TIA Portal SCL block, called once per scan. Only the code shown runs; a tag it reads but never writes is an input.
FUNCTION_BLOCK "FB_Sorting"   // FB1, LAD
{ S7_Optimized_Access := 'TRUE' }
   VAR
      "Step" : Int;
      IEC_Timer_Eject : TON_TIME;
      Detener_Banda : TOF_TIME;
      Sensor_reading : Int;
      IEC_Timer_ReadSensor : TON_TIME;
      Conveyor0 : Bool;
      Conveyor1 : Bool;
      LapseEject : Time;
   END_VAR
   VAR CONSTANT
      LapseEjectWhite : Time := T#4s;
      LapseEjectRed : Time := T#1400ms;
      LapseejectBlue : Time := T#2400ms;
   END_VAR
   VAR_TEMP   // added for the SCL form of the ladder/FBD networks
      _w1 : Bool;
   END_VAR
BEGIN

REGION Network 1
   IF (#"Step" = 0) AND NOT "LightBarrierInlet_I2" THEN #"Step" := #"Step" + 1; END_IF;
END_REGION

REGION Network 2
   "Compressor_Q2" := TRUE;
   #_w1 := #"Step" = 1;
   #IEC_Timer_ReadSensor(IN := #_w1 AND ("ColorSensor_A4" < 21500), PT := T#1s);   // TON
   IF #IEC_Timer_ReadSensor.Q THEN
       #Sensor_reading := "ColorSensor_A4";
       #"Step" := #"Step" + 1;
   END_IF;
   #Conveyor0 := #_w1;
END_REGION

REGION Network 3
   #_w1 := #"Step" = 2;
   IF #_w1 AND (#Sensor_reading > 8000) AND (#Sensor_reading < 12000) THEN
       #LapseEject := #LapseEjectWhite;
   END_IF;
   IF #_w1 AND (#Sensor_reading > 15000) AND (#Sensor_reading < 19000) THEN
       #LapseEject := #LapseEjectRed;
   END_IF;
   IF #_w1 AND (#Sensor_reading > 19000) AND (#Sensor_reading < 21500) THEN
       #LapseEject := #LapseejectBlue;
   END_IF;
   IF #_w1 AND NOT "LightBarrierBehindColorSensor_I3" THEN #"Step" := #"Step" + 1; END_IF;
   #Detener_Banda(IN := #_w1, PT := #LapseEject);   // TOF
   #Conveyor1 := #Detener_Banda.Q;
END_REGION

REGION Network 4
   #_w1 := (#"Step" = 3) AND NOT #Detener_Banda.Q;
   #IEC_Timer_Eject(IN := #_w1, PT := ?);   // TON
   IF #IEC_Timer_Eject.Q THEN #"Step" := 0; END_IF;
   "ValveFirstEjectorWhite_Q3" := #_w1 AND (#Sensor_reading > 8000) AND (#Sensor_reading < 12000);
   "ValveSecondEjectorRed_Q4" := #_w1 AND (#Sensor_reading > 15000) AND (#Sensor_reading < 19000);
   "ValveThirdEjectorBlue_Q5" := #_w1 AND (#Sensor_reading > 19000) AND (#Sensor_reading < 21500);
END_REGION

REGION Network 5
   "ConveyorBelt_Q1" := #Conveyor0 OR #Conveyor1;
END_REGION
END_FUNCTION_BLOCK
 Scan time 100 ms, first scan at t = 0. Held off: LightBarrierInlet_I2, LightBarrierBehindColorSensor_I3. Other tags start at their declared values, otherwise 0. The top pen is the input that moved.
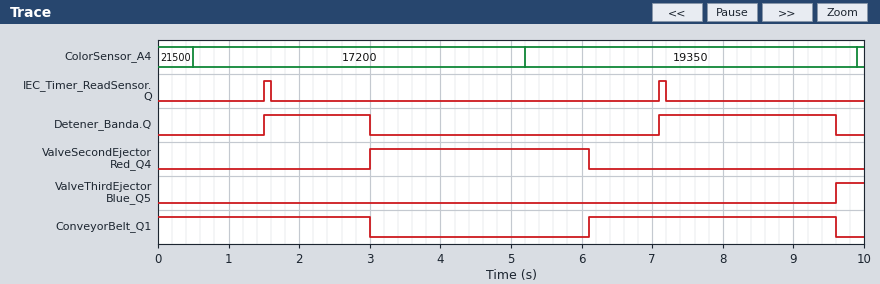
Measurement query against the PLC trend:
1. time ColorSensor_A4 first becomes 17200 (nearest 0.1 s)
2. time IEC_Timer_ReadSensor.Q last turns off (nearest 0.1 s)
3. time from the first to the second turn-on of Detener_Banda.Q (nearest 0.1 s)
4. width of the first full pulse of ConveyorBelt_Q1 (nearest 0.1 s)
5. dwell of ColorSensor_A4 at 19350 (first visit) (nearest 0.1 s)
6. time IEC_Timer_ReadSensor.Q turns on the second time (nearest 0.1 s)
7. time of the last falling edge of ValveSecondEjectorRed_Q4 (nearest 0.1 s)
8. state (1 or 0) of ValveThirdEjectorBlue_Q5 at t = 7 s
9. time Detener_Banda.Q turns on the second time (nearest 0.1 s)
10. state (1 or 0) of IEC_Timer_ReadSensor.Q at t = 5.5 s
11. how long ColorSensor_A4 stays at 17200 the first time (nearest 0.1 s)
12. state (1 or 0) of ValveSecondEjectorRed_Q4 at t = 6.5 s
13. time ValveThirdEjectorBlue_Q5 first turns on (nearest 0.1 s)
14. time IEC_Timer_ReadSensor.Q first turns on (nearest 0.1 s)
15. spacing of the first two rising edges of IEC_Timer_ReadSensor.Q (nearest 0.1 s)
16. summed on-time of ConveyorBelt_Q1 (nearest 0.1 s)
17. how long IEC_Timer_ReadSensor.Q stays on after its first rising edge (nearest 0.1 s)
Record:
0.5 s
7.2 s
5.6 s
3.5 s
4.7 s
7.1 s
6.1 s
0
7.1 s
0
4.7 s
0
9.6 s
1.5 s
5.6 s
6.5 s
0.1 s
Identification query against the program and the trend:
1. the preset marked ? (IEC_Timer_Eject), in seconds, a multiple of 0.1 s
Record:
3.0 s
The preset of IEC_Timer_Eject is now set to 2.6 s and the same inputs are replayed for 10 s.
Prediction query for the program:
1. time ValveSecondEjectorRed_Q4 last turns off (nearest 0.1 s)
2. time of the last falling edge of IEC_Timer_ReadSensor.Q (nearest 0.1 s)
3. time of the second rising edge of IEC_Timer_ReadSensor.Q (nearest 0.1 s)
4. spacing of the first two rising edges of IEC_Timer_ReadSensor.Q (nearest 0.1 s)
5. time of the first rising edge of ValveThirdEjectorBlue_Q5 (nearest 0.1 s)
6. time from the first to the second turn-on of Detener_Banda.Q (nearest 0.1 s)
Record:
5.7 s
6.8 s
6.7 s
5.2 s
9.2 s
5.2 s
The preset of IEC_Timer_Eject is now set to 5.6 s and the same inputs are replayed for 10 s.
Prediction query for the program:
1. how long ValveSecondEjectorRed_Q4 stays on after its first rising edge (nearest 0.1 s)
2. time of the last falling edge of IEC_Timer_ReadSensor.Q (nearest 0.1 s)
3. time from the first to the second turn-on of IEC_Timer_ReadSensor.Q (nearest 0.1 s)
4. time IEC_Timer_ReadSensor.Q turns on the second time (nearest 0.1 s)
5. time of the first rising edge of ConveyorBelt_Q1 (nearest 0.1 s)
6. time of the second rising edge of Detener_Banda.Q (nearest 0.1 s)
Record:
5.7 s
9.8 s
8.2 s
9.7 s
8.7 s
9.7 s
